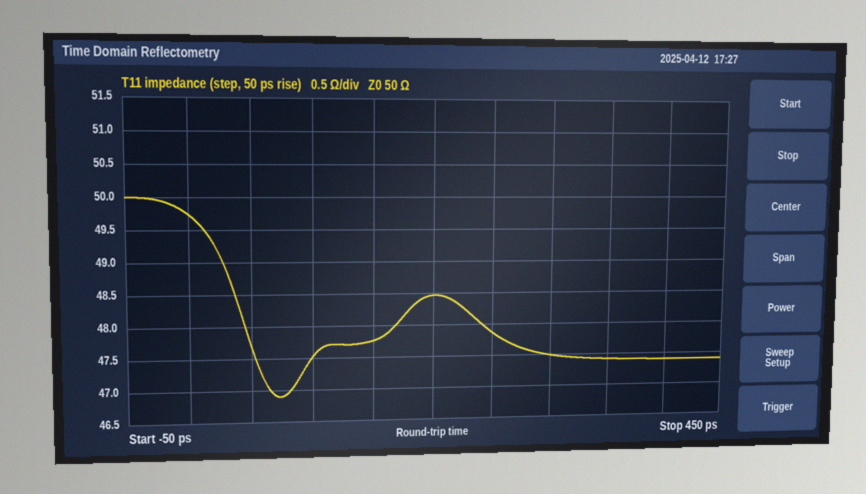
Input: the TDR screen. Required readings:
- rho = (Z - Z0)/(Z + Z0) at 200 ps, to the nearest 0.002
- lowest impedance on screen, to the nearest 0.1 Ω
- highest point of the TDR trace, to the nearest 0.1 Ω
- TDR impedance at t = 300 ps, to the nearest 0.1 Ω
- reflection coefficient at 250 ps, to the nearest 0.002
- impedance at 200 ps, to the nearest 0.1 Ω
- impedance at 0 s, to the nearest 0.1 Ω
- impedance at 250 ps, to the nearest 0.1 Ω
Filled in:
-0.016
46.9 Ω
50.0 Ω
47.5 Ω
-0.022
48.5 Ω
49.7 Ω
47.9 Ω
